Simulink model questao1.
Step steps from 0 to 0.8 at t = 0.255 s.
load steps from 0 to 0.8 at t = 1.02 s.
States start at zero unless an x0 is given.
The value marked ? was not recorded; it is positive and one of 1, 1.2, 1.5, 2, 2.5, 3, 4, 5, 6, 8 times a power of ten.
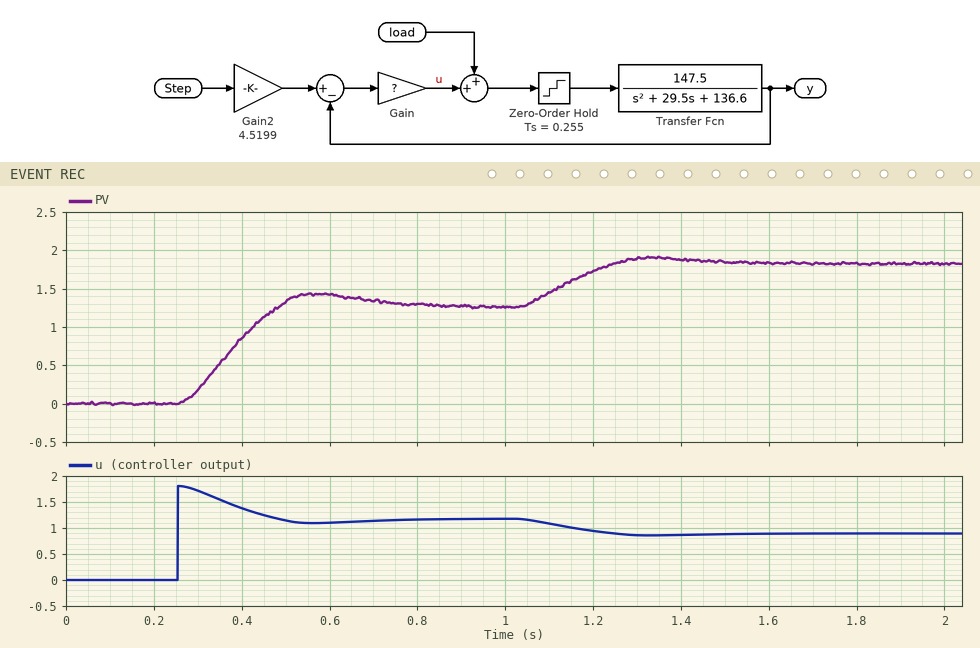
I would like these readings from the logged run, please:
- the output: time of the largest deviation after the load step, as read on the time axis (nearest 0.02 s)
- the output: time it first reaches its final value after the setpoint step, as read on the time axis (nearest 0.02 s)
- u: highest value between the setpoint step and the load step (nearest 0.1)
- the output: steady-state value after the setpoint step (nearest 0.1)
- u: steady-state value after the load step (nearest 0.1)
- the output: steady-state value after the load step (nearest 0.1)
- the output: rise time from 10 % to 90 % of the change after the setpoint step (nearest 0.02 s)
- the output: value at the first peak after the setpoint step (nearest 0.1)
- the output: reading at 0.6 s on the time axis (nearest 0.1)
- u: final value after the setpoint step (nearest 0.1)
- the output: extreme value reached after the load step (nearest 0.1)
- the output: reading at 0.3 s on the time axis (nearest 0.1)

1.32 s
0.48 s
1.8
1.3
0.9
1.8
0.16 s
1.4
1.4
1.2
1.9
0.2
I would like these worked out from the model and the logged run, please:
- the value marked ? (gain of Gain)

0.5
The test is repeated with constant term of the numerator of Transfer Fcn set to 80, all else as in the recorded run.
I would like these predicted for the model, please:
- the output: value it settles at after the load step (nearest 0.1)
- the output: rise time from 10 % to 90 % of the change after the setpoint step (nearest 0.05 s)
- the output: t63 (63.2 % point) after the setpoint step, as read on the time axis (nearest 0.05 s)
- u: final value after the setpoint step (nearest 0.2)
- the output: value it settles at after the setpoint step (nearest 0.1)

1.2
0.20 s
0.40 s
1.4
0.8
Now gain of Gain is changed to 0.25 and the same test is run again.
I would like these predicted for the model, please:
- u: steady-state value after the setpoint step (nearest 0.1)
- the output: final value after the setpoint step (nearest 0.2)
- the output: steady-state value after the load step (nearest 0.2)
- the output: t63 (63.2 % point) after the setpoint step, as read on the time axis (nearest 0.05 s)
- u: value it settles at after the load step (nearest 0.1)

0.7
0.8
1.4
0.40 s
0.5
